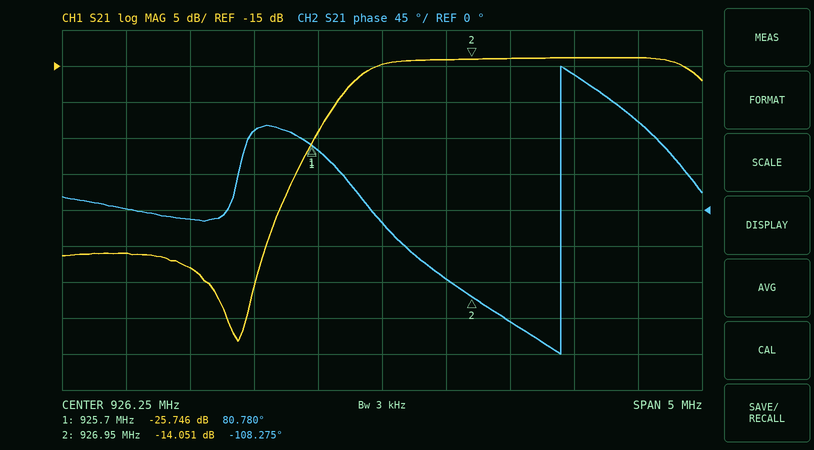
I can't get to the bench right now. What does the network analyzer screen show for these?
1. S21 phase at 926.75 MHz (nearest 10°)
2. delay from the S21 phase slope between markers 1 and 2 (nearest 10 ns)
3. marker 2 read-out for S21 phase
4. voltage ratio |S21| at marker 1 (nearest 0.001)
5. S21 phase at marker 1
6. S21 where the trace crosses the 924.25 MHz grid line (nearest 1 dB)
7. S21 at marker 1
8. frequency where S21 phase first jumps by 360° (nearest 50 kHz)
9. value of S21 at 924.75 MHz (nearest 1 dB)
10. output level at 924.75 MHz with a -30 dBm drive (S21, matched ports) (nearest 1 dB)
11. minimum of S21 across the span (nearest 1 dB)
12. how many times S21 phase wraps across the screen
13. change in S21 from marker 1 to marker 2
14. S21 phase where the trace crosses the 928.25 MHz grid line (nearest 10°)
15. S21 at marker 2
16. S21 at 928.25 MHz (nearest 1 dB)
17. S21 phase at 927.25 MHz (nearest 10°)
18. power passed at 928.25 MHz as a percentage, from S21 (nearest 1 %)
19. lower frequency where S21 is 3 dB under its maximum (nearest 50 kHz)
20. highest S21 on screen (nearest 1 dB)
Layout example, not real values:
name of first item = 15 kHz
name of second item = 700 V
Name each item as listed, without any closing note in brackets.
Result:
S21 phase at 926.75 MHz = -90°
delay from the S21 phase slope between markers 1 and 2 = 420 ns
marker 2 read-out for S21 phase = -108.275°
voltage ratio |S21| at marker 1 = 0.052
S21 phase at marker 1 = 80.780°
S21 where the trace crosses the 924.25 MHz grid line = -41 dB
S21 at marker 1 = -25.746 dB
frequency where S21 phase first jumps by 360° = 927.65 MHz
value of S21 at 924.75 MHz = -43 dB
output level at 924.75 MHz with a -30 dBm drive (S21, matched ports) = -73 dBm
minimum of S21 across the span = -53 dB
how many times S21 phase wraps across the screen = 1
change in S21 from marker 1 to marker 2 = 11.695 dB
S21 phase where the trace crosses the 928.25 MHz grid line = 110°
S21 at marker 2 = -14.051 dB
S21 at 928.25 MHz = -14 dB
S21 phase at 927.25 MHz = -140°
power passed at 928.25 MHz as a percentage, from S21 = 4 %
lower frequency where S21 is 3 dB under its maximum = 926.05 MHz
highest S21 on screen = -14 dB
